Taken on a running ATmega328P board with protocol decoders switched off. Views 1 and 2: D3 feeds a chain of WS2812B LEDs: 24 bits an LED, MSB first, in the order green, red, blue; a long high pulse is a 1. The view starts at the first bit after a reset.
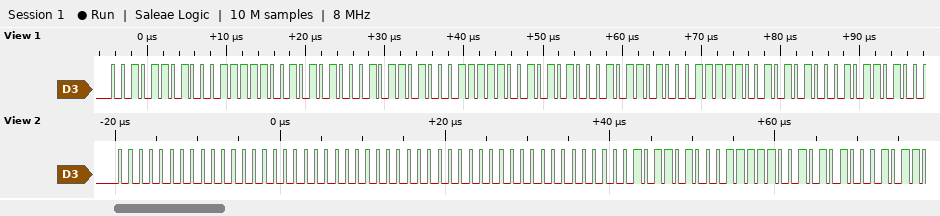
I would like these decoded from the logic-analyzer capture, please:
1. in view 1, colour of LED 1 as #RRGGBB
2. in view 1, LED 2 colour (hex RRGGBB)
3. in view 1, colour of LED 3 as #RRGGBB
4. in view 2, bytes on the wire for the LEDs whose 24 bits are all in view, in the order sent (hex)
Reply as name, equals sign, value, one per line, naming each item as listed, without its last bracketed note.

in view 1, colour of LED 1 as #RRGGBB = #1F2D2A
in view 1, LED 2 colour = #1F2D2A
in view 1, colour of LED 3 as #RRGGBB = #1F2D2A
in view 2, bytes on the wire for the LEDs whose 24 bits are all in view, in the order sent = 00 00 00 00 00 00 2D 1F 2A
